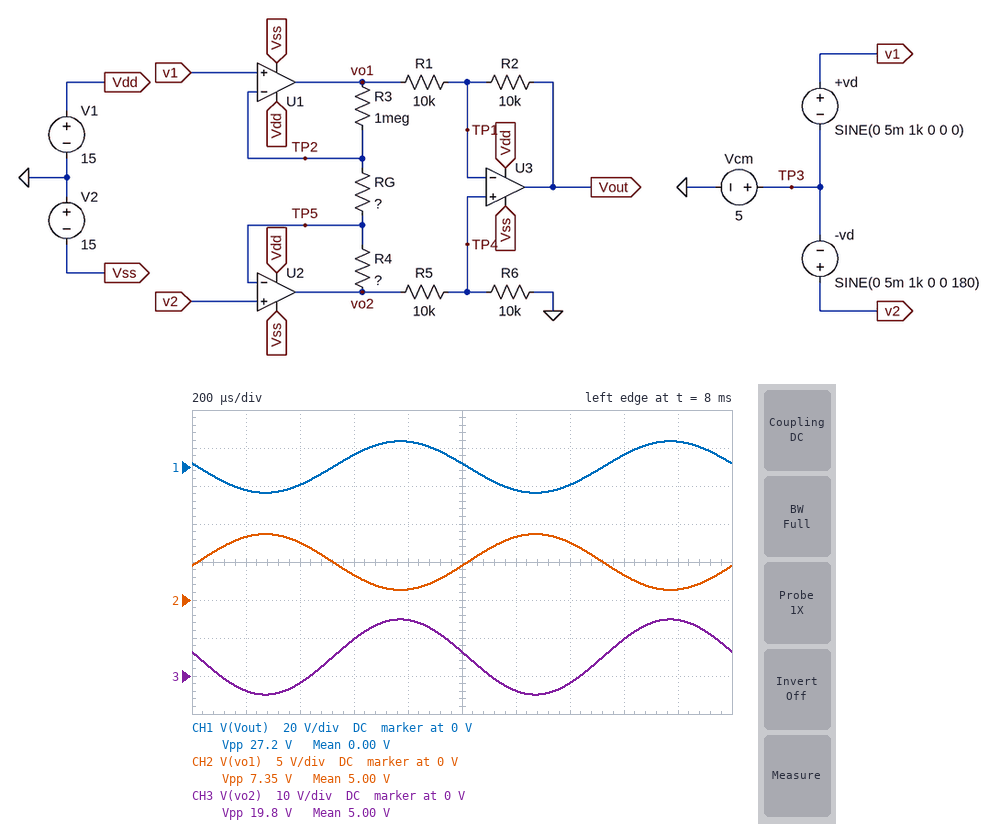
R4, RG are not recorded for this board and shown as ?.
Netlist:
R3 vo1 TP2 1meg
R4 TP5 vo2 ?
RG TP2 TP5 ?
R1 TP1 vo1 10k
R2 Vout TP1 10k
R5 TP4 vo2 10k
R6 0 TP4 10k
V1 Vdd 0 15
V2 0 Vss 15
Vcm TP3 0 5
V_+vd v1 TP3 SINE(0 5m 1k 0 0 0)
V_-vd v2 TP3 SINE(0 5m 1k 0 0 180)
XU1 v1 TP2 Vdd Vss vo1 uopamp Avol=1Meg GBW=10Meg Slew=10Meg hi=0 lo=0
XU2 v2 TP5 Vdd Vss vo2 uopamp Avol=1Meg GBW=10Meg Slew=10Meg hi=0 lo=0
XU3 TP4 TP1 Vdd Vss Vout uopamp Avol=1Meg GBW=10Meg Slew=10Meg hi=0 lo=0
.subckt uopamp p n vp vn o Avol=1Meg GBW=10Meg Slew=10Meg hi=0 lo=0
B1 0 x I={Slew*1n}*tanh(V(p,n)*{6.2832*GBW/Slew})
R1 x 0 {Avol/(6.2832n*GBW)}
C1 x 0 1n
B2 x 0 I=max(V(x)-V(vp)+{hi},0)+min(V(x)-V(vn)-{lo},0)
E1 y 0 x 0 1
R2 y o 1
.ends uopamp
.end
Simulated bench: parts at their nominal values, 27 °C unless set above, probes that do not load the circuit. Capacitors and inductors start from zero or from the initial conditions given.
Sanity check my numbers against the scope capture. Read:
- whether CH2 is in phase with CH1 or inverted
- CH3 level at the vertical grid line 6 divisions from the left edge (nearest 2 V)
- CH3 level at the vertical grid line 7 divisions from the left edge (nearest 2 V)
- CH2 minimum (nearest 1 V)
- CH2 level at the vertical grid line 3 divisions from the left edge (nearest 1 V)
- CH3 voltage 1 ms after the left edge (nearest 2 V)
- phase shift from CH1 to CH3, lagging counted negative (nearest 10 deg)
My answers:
inverted
-4 V
-2 V
1 V
3 V
6 V
0 deg
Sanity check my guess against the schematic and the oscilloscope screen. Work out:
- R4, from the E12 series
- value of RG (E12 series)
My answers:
2.7 MΩ
2.7 kΩ
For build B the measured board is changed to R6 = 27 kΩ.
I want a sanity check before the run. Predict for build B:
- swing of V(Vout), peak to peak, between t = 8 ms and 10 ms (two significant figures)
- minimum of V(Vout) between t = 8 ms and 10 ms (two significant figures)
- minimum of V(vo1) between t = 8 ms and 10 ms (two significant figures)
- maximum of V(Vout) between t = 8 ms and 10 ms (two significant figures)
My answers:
30 V
-15 V
1.3 V
15 V
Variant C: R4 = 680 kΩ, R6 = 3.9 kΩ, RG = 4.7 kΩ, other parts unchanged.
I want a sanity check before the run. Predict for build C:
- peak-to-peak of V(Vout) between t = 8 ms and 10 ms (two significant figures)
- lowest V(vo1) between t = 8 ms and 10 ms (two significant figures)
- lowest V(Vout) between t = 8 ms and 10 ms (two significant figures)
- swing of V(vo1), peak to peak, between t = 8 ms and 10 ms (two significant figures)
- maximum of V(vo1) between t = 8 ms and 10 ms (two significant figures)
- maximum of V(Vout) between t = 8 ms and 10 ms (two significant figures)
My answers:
5.9 V
2.9 V
-5.1 V
4.3 V
7.1 V
750 mV
